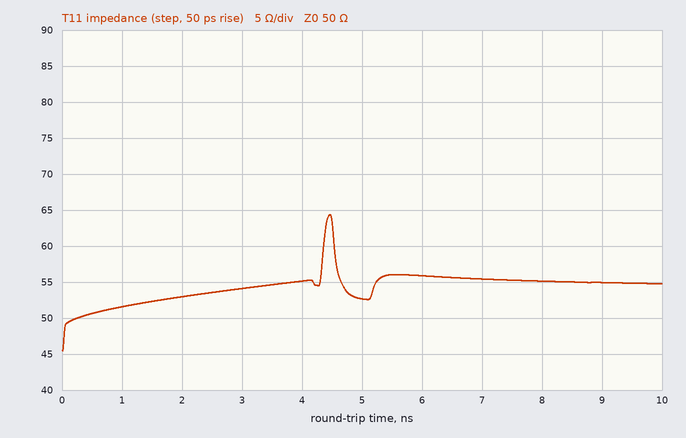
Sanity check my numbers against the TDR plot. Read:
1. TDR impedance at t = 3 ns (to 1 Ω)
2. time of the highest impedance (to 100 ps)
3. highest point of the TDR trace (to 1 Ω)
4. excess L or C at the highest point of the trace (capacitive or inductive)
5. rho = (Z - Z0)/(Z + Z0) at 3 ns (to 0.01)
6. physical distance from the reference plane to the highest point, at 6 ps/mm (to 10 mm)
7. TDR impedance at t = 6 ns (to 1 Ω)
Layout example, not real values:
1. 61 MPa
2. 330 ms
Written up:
1. 54 Ω
2. 4.5 ns
3. 64 Ω
4. inductive
5. +0.04
6. 370 mm
7. 56 Ω
